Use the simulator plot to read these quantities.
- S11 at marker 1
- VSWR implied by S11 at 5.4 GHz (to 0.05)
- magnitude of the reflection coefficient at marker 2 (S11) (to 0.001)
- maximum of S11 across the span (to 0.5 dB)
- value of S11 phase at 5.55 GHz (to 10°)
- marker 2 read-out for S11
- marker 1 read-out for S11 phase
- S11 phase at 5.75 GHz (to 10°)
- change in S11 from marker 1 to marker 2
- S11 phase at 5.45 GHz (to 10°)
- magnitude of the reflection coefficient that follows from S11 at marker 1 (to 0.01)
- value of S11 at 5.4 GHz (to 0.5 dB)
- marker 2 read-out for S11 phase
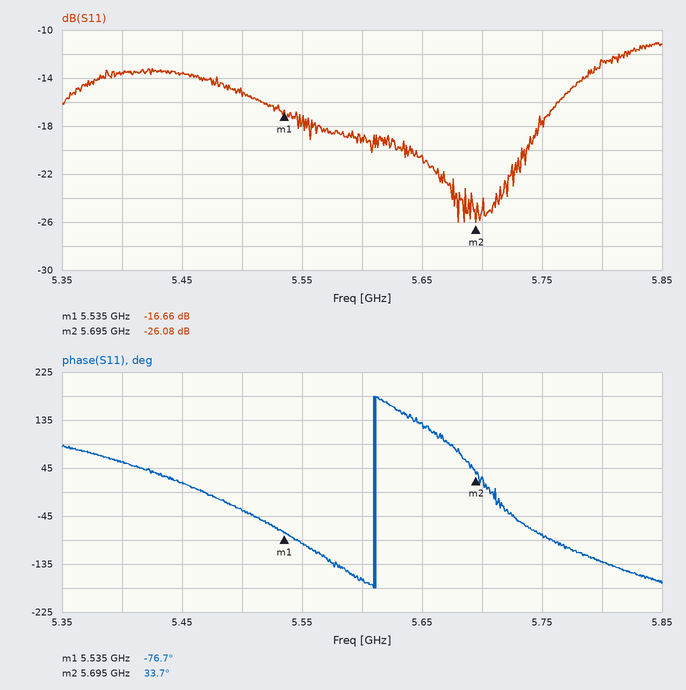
-16.66 dB
1.55
0.050
-11.0 dB
-100°
-26.08 dB
-76.7°
-80°
-9.42 dB
20°
0.15
-13.5 dB
33.7°
